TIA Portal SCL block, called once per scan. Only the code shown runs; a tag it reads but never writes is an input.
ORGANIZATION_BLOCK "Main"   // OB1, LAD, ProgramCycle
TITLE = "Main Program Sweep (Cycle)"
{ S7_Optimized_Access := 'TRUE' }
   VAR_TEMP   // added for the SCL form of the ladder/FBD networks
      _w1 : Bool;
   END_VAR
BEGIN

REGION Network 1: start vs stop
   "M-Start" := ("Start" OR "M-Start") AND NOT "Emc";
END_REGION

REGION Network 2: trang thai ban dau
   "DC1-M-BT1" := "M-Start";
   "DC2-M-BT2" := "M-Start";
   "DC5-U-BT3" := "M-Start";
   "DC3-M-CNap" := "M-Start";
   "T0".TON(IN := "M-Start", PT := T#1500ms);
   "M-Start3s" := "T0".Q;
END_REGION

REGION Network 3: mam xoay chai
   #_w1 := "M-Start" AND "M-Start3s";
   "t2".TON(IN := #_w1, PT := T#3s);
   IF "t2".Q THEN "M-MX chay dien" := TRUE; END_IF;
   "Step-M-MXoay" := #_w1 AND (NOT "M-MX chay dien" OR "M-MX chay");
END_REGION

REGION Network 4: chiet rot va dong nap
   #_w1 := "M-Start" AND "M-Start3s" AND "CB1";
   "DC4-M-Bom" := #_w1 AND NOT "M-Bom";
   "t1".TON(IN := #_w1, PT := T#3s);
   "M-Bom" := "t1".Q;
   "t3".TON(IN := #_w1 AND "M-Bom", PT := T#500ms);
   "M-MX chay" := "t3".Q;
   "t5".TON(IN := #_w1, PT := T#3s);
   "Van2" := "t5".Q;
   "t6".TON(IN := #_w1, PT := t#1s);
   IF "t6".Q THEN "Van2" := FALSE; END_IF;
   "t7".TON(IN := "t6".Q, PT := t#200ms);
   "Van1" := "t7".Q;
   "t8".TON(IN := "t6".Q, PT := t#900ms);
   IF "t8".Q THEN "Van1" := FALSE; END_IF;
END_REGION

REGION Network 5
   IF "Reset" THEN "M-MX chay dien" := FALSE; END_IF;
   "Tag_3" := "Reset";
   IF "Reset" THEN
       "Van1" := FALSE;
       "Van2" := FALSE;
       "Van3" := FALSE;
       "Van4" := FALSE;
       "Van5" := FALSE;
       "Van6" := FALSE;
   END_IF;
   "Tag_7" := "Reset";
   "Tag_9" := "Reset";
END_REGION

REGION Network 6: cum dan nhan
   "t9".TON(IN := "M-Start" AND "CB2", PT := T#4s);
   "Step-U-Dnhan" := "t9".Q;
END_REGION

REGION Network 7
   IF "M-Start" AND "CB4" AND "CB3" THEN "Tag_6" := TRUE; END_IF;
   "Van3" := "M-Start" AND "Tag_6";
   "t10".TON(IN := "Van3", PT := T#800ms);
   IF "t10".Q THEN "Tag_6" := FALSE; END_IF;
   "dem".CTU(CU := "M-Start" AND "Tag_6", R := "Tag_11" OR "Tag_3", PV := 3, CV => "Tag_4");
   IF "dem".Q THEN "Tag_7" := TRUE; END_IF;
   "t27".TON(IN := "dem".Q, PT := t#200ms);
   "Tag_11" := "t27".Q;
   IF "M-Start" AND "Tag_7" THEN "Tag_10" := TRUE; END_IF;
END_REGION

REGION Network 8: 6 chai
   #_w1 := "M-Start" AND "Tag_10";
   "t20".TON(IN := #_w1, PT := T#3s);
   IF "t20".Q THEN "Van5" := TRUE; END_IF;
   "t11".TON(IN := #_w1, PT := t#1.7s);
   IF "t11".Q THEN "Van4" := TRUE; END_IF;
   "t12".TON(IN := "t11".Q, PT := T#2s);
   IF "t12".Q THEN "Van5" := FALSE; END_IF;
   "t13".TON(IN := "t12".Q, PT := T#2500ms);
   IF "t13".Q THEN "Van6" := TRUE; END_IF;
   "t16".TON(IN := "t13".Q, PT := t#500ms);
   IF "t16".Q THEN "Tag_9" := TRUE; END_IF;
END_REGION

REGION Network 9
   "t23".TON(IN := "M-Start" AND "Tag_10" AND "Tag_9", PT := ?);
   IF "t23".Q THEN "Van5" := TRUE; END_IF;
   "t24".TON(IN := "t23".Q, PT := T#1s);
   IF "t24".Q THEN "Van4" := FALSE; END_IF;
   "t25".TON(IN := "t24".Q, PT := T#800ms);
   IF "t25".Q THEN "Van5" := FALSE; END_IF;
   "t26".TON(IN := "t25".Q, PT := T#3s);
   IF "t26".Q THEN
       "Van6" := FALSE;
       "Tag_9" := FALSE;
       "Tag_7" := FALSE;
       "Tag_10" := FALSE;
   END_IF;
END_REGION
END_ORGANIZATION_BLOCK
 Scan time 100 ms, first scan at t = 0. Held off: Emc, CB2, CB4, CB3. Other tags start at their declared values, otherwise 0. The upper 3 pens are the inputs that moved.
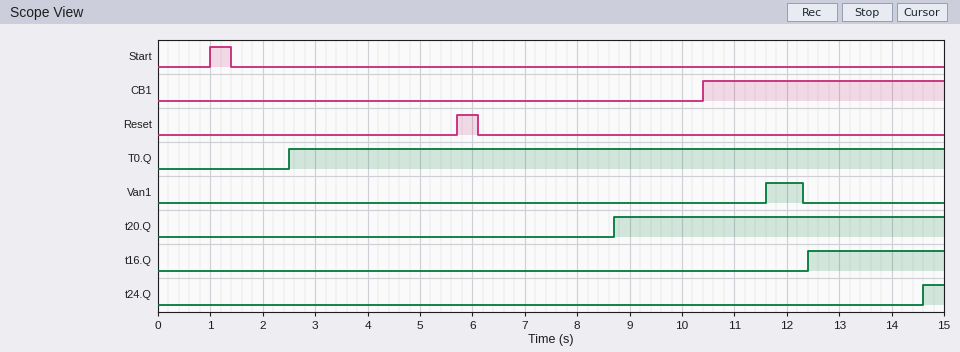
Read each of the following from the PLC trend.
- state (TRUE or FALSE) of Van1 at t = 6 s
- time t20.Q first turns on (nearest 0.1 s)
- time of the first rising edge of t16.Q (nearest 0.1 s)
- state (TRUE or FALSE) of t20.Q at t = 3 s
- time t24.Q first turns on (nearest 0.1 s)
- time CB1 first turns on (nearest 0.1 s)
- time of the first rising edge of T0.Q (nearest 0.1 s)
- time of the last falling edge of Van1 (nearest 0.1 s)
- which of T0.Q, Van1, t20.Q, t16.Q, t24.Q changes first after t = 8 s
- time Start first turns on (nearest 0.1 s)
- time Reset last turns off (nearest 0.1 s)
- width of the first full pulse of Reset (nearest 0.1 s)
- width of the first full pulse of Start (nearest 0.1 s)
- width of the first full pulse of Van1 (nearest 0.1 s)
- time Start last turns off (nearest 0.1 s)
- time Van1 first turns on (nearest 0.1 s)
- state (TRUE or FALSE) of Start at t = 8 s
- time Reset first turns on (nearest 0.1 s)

FALSE
8.7 s
12.4 s
FALSE
14.6 s
10.4 s
2.5 s
12.3 s
t20.Q
1.0 s
6.1 s
0.4 s
0.4 s
0.7 s
1.4 s
11.6 s
FALSE
5.7 s
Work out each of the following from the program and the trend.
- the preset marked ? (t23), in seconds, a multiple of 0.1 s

1.2 s
